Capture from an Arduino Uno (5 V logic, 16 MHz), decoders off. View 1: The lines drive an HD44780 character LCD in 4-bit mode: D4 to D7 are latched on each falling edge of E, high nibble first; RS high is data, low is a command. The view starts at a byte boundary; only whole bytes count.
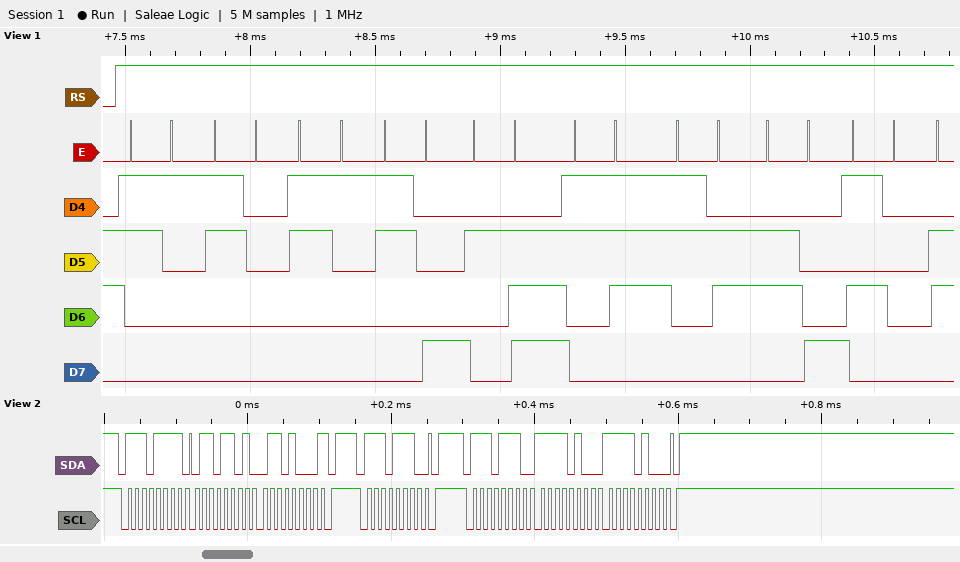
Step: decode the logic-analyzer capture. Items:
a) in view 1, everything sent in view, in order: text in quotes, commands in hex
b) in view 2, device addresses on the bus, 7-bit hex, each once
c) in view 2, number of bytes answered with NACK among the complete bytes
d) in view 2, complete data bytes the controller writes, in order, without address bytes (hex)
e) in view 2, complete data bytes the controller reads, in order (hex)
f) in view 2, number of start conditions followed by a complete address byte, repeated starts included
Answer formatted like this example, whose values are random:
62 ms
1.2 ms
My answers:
"1018.76hP"
0x77
1
F4 F4
6D 68
3
